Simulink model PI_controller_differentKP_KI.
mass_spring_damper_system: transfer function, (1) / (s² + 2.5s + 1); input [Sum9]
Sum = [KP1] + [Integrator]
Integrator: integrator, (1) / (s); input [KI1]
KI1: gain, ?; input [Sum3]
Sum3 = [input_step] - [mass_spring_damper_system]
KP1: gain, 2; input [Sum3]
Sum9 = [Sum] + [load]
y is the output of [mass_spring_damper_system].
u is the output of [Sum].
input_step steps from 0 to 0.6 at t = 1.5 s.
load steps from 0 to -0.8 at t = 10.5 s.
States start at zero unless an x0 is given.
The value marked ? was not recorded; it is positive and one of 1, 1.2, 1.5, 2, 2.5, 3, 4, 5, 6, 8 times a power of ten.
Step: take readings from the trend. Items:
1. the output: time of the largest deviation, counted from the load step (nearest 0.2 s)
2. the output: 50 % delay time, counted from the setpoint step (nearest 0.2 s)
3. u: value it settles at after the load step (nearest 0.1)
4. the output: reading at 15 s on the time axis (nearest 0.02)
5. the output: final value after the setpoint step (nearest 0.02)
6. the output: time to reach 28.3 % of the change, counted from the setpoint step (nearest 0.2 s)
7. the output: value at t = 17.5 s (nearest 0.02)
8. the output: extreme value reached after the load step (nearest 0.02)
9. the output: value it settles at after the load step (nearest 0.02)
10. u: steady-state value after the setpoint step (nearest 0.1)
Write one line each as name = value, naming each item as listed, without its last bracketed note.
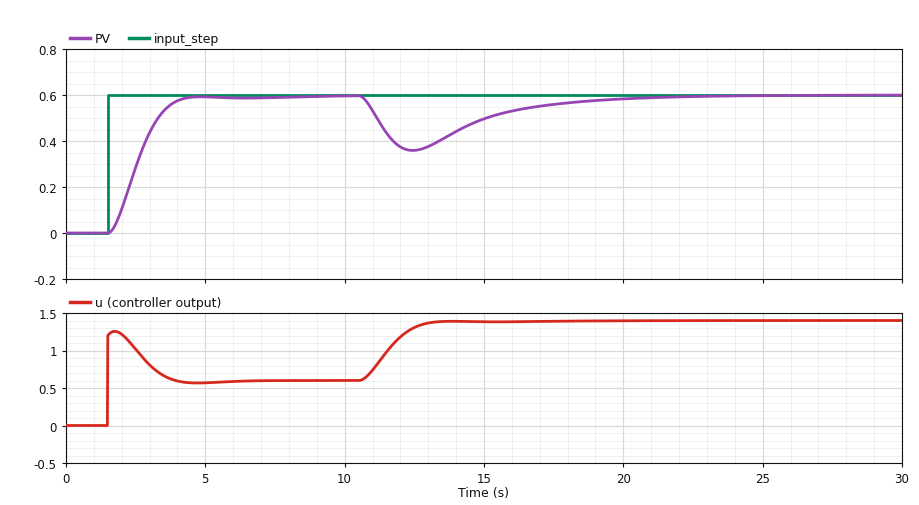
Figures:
the output: time of the largest deviation, counted from the load step = 2.0 s
the output: 50 % delay time, counted from the setpoint step = 1.0 s
u: value it settles at after the load step = 1.4
the output: reading at 15 s on the time axis = 0.50
the output: final value after the setpoint step = 0.60
the output: time to reach 28.3 % of the change, counted from the setpoint step = 0.6 s
the output: value at t = 17.5 s = 0.56
the output: extreme value reached after the load step = 0.36
the output: value it settles at after the load step = 0.60
u: steady-state value after the setpoint step = 0.6
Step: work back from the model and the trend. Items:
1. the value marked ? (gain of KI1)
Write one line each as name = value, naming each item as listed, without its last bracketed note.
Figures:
the value marked ? = 0.8
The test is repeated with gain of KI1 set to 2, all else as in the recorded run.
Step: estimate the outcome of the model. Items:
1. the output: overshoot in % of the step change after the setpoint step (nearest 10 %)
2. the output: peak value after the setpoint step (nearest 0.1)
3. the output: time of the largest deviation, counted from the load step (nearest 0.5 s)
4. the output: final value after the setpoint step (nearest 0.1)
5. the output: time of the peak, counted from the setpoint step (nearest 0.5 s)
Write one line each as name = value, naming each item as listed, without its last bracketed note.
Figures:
the output: overshoot in % of the step change after the setpoint step = 30 %
the output: peak value after the setpoint step = 0.8
the output: time of the largest deviation, counted from the load step = 1.5 s
the output: final value after the setpoint step = 0.6
the output: time of the peak, counted from the setpoint step = 2.5 s
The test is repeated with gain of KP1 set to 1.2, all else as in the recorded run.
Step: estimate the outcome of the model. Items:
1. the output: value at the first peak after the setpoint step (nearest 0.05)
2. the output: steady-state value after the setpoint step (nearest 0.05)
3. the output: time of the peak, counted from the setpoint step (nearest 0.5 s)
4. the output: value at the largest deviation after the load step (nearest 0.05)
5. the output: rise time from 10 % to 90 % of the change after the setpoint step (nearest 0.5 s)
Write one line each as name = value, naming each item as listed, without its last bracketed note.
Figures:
the output: value at the first peak after the setpoint step = 0.65
the output: steady-state value after the setpoint step = 0.60
the output: time of the peak, counted from the setpoint step = 4.5 s
the output: value at the largest deviation after the load step = 0.30
the output: rise time from 10 % to 90 % of the change after the setpoint step = 2.0 s
